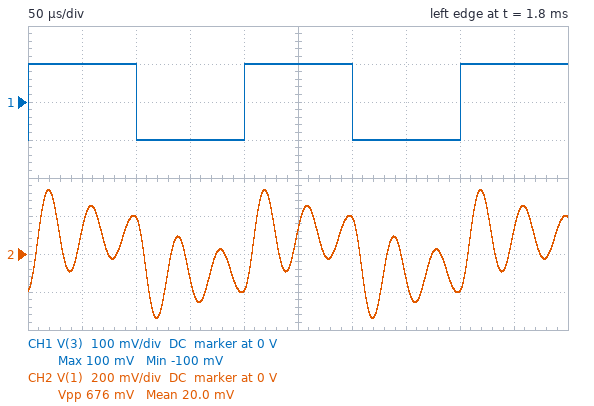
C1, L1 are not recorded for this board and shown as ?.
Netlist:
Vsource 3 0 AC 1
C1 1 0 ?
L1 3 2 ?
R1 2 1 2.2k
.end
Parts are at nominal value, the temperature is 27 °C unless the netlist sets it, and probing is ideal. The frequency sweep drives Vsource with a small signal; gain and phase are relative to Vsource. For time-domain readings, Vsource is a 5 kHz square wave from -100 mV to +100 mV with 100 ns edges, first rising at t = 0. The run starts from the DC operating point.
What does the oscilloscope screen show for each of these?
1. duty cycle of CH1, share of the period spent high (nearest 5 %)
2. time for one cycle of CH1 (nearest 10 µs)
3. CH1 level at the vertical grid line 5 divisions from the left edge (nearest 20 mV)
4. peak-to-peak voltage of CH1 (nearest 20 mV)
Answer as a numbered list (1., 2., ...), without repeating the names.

1. 50 %
2. 200 µs
3. 100 mV
4. 200 mV
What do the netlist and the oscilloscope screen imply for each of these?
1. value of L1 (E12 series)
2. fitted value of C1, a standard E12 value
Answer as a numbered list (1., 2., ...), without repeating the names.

1. 100 mH
2. 390 pF
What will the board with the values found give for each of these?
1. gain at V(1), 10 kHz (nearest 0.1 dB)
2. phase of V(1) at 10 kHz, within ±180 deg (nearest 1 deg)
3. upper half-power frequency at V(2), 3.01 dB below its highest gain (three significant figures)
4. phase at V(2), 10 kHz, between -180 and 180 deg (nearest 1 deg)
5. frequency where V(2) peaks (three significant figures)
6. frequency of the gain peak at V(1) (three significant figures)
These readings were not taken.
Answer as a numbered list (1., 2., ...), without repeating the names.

1. 1.4 dB
2. -4 deg
3. 27.1 kHz
4. -1 deg
5. 25.4 kHz
6. 25.4 kHz
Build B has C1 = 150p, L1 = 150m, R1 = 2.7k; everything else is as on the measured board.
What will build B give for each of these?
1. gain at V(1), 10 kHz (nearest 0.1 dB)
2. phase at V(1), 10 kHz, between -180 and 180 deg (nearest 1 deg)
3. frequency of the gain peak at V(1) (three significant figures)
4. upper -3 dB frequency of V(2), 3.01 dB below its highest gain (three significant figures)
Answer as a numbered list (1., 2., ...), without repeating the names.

1. 0.8 dB
2. -2 deg
3. 33.5 kHz
4. 34.9 kHz
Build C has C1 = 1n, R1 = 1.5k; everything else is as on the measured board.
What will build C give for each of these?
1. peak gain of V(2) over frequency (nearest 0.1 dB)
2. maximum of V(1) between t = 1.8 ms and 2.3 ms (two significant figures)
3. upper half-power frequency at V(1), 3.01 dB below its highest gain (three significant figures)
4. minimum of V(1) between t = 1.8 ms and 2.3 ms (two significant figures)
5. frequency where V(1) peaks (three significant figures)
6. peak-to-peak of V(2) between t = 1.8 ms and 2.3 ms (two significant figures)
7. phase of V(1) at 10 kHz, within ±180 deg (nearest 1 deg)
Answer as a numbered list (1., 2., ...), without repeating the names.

1. 16.6 dB
2. 350 mV
3. 17.0 kHz
4. -350 mV
5. 15.8 kHz
6. 710 mV
7. -9 deg
